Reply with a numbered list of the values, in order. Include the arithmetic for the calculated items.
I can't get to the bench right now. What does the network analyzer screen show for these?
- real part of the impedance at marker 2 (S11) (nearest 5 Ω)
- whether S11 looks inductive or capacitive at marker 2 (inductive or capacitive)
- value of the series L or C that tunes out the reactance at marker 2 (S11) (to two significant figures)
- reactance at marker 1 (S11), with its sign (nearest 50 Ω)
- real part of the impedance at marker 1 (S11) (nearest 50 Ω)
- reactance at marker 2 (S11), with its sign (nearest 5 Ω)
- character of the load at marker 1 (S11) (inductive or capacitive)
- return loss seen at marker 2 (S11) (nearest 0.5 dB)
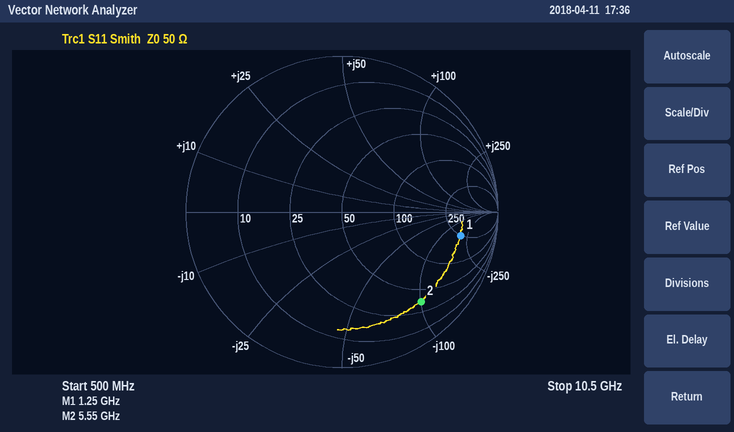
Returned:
1. 35 Ω
2. capacitive
3. L = 100 Ω/(2π × 5.55 GHz) ≈ 2.9 nH
4. -200 Ω
5. 250 Ω
6. -100 Ω
7. capacitive
8. 2.5 dB
